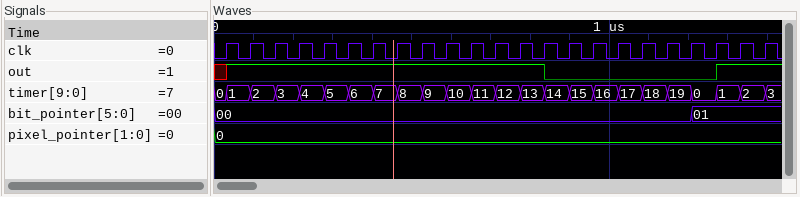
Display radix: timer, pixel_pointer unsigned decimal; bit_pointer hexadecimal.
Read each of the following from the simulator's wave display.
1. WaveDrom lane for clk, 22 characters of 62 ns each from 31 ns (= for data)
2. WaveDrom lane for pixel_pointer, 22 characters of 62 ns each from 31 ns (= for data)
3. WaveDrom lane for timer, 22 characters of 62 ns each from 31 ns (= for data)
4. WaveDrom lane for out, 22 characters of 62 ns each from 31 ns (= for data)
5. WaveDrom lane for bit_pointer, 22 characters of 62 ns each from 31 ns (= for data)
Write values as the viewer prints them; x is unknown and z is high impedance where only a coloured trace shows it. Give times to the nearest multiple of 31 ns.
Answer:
{name: 'clk', wave: 'p.....................'}
{name: 'pixel_pointer', wave: '=.....................', data: '0'}
{name: 'timer', wave: '======================', data: '1 2 3 4 5 6 7 8 9 10 11 12 13 14 15 16 17 18 19 0 1 2'}
{name: 'out', wave: '1............0......1.'}
{name: 'bit_pointer', wave: '=..................=..', data: '00 01'}
